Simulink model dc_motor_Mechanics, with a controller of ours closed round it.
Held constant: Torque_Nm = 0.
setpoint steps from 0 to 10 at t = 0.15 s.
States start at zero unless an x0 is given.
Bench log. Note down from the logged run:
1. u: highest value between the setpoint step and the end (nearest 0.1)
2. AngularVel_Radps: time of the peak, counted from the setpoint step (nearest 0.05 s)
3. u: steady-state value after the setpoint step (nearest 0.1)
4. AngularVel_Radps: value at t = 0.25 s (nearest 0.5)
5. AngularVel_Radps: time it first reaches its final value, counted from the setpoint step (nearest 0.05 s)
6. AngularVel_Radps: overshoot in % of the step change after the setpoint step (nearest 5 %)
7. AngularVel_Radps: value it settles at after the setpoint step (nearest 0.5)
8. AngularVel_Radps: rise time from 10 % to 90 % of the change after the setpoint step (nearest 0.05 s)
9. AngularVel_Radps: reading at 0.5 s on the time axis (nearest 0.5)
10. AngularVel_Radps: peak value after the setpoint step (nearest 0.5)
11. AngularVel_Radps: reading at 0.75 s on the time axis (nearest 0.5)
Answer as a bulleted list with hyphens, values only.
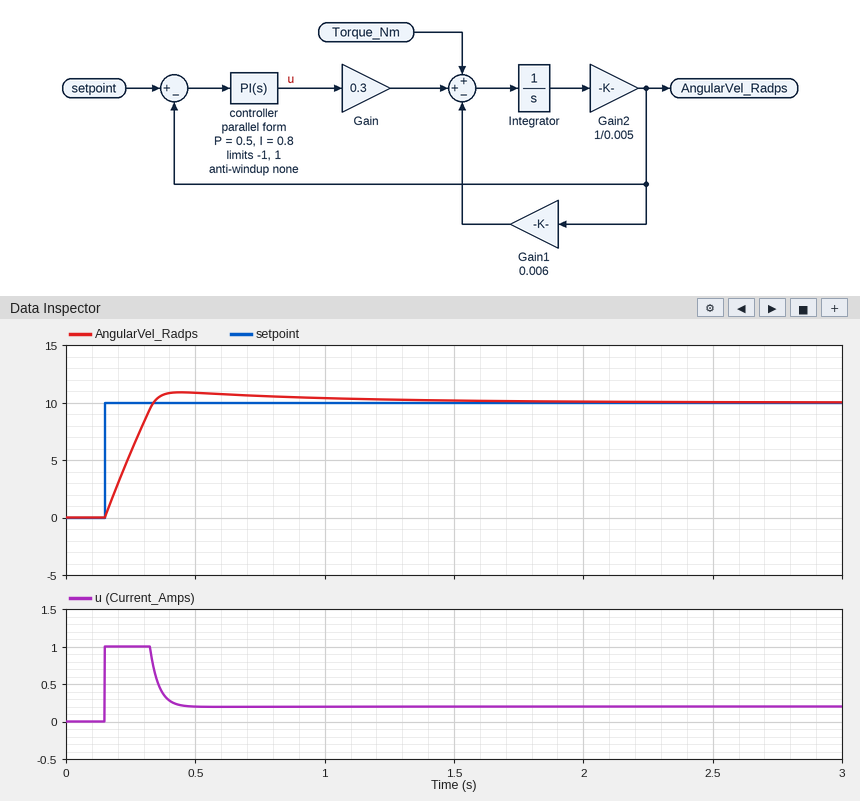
- 1.0
- 0.30 s
- 0.2
- 5.5
- 0.20 s
- 10 %
- 10.0
- 0.15 s
- 11.0
- 11.0
- 10.5
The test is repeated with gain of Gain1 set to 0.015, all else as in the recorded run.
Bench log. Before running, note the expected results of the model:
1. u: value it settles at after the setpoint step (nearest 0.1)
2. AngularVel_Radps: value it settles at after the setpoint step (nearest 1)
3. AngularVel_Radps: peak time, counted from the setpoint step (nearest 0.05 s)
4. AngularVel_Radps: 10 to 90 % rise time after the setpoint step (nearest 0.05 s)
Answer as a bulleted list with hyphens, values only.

- 0.5
- 10
- 0.35 s
- 0.20 s
